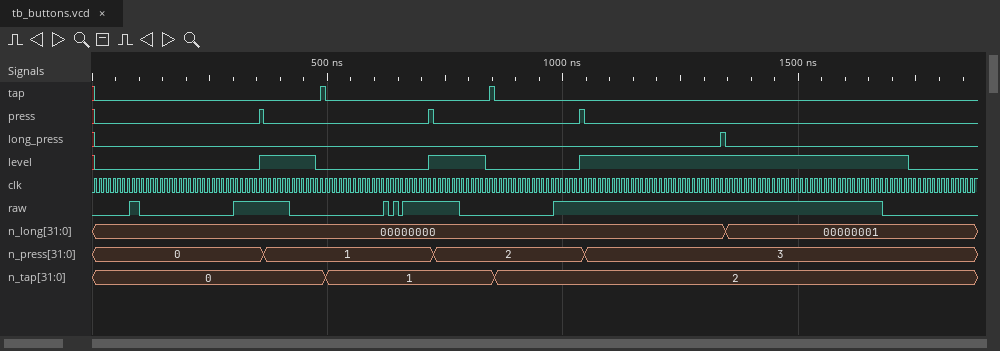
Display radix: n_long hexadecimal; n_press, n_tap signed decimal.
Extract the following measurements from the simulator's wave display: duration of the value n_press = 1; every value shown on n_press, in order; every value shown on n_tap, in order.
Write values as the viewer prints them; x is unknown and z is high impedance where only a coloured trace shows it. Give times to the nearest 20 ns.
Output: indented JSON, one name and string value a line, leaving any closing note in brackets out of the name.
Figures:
{
  "duration of the value n_press = 1": "360 ns",
  "every value shown on n_press, in order": "0, 1, 2, 3",
  "every value shown on n_tap, in order": "0, 1, 2"
}
